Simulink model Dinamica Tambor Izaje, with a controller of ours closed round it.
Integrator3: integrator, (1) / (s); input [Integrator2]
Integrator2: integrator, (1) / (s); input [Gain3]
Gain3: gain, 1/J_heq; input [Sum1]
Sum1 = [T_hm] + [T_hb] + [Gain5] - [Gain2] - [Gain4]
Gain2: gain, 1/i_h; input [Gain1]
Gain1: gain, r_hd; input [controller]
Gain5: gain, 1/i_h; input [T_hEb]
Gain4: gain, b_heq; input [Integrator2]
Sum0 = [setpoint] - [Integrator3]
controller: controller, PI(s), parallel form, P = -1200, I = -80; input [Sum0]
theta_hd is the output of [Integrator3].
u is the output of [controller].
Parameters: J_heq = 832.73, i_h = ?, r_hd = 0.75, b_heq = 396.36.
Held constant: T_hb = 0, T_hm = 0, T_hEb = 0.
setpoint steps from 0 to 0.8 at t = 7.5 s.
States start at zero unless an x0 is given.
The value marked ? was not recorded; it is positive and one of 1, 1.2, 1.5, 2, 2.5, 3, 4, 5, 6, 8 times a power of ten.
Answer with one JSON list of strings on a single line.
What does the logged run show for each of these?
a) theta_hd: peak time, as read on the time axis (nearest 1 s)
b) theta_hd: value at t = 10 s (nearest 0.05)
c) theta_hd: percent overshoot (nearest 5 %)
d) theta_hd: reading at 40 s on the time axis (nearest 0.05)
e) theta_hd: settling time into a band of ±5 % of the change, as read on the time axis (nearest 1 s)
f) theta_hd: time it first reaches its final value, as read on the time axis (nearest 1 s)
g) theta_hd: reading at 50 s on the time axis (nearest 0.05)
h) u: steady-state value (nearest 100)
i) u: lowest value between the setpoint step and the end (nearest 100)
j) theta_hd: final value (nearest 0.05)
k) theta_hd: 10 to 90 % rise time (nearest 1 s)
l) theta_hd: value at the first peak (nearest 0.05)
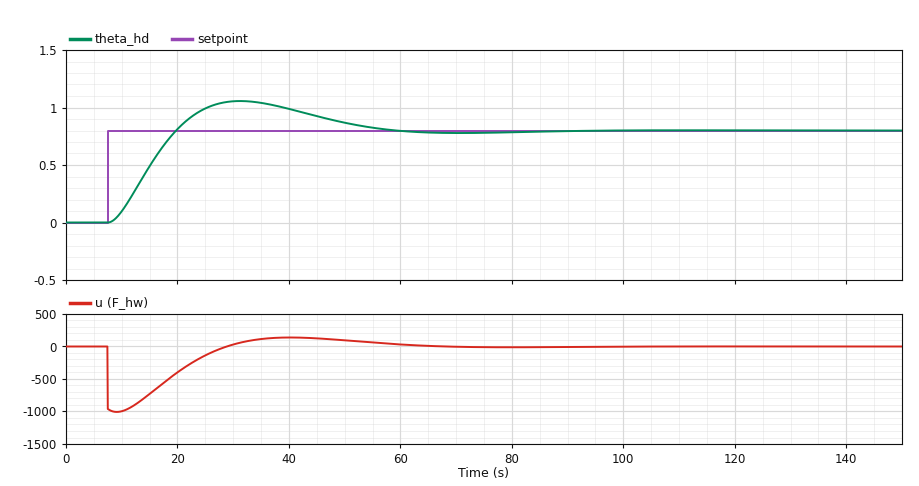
["31 s", "0.10", "30 %", "1.00", "53 s", "20 s", "0.85", "0", "-1000", "0.80", "9 s", "1.05"]
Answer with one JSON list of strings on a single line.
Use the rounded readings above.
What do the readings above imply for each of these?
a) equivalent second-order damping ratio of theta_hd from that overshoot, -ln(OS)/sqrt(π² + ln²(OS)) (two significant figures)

["0.36"]
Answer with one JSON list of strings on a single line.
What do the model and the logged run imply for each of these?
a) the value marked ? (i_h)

["20"]
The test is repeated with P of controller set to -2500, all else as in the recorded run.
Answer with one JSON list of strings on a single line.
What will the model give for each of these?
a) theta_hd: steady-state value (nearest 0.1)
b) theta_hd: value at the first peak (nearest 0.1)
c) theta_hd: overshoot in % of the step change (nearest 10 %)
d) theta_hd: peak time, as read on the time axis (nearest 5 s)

["0.8", "0.9", "20 %", "20 s"]
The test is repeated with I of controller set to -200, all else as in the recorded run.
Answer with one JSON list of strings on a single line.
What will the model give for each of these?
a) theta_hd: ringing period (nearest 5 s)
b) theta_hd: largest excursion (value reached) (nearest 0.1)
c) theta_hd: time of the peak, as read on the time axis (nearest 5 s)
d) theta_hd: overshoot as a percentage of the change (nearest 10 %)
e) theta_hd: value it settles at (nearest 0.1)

["45 s", "1.3", "25 s", "60 %", "0.8"]
